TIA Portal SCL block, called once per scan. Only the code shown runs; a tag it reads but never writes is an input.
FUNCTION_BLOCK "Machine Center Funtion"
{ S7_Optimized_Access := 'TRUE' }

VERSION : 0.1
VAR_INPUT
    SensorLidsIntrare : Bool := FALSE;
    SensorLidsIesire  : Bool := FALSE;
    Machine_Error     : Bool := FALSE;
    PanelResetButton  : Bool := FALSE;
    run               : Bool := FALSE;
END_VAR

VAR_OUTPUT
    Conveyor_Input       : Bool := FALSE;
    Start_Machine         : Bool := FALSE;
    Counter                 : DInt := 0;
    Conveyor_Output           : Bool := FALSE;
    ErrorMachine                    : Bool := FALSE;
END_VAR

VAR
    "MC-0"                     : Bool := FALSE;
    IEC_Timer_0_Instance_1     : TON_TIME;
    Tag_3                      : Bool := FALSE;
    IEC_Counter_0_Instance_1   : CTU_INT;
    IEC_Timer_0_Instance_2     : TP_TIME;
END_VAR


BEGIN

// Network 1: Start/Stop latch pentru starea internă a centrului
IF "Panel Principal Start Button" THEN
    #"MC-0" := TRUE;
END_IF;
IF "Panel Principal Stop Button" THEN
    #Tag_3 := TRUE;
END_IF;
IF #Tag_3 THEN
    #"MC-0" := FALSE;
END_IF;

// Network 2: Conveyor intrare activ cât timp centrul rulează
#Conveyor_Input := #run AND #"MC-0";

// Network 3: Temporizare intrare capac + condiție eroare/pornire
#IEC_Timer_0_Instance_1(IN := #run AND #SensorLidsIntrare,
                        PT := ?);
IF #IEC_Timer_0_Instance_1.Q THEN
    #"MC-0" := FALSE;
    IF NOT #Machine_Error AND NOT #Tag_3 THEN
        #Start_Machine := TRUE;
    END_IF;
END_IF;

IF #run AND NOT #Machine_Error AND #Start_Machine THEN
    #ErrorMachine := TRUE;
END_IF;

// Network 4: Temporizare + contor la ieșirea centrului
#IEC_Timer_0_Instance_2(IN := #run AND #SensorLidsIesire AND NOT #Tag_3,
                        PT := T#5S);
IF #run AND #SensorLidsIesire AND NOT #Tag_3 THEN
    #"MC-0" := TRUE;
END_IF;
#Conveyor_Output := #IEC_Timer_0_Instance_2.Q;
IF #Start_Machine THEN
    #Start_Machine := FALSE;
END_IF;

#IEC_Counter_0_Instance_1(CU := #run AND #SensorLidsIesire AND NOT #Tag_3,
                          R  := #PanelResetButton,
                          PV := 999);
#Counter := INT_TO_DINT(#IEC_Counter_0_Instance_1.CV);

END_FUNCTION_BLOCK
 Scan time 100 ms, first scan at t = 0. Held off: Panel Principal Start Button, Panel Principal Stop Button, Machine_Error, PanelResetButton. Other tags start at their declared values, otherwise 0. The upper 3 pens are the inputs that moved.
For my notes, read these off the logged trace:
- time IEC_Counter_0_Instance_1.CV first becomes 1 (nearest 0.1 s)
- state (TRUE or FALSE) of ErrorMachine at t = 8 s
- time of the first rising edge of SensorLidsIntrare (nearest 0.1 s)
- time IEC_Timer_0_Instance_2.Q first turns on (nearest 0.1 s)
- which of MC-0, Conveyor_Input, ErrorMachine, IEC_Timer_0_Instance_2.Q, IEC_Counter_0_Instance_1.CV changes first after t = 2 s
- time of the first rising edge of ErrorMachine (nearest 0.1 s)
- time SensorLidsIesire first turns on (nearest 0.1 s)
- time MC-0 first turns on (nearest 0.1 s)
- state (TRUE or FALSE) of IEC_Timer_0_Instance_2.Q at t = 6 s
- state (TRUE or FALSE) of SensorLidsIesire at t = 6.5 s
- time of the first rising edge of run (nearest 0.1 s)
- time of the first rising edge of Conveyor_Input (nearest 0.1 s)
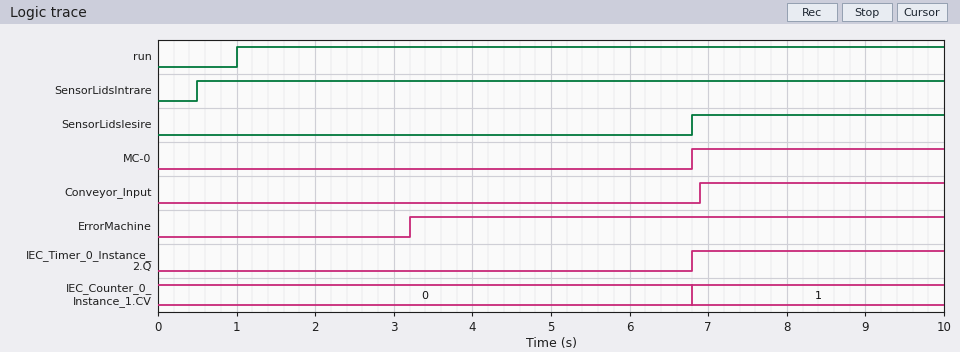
6.8 s
TRUE
0.5 s
6.8 s
ErrorMachine
3.2 s
6.8 s
6.8 s
FALSE
FALSE
1.0 s
6.9 s
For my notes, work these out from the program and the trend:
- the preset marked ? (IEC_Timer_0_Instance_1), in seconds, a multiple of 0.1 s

2.2 s
